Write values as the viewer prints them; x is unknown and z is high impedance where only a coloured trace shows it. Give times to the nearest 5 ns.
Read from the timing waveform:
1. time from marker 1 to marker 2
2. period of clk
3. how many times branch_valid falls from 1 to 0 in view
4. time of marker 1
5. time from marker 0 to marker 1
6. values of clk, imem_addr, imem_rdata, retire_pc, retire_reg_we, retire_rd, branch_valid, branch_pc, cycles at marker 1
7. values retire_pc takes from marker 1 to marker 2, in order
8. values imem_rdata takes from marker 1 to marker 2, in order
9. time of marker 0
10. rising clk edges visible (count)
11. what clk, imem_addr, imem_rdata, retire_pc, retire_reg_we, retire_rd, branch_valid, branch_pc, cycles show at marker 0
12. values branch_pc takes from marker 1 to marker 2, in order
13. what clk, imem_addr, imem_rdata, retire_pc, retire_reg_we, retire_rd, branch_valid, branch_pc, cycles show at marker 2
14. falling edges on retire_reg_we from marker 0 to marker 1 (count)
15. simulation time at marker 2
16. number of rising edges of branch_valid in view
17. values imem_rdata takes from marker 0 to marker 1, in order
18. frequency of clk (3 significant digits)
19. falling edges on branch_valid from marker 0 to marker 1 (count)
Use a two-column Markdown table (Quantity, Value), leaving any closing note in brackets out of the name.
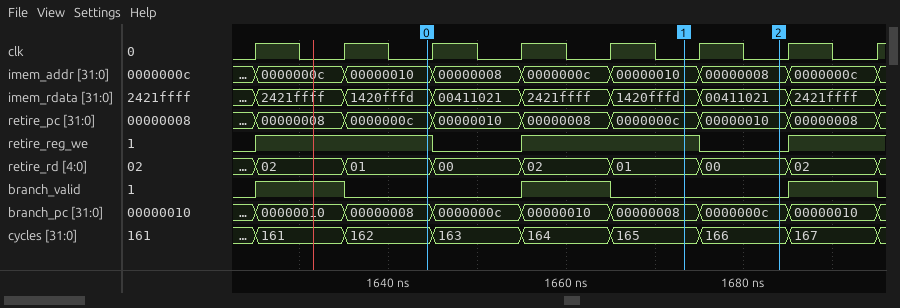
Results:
| Quantity | Value |
|---|---|
| time from marker 1 to marker 2 | 10 ns |
| period of clk | 10 ns |
| how many times branch_valid falls from 1 to 0 in view | 3 |
| time of marker 1 | 1675 ns |
| time from marker 0 to marker 1 | 30 ns |
| values of clk, imem_addr, imem_rdata, retire_pc, retire_reg_we, retire_rd, branch_valid, branch_pc, cycles at marker 1 | clk=0, imem_addr=00000010, imem_rdata=1420fffd, retire_pc=0000000c, retire_reg_we=1, retire_rd=01, branch_valid=0, branch_pc=00000008, cycles=165 |
| values retire_pc takes from marker 1 to marker 2, in order | 0000000c, 00000010 |
| values imem_rdata takes from marker 1 to marker 2, in order | 1420fffd, 00411021 |
| time of marker 0 | 1645 ns |
| rising clk edges visible | 8 |
| what clk, imem_addr, imem_rdata, retire_pc, retire_reg_we, retire_rd, branch_valid, branch_pc, cycles show at marker 0 | clk=0, imem_addr=00000010, imem_rdata=1420fffd, retire_pc=0000000c, retire_reg_we=1, retire_rd=01, branch_valid=0, branch_pc=00000008, cycles=162 |
| values branch_pc takes from marker 1 to marker 2, in order | 00000008, 0000000c |
| what clk, imem_addr, imem_rdata, retire_pc, retire_reg_we, retire_rd, branch_valid, branch_pc, cycles show at marker 2 | clk=0, imem_addr=00000008, imem_rdata=00411021, retire_pc=00000010, retire_reg_we=0, retire_rd=00, branch_valid=0, branch_pc=0000000c, cycles=166 |
| falling edges on retire_reg_we from marker 0 to marker 1 | 1 |
| simulation time at marker 2 | 1685 ns |
| number of rising edges of branch_valid in view | 3 |
| values imem_rdata takes from marker 0 to marker 1, in order | 1420fffd, 00411021, 2421ffff, 1420fffd |
| frequency of clk | 100 MHz |
| falling edges on branch_valid from marker 0 to marker 1 | 1 |
